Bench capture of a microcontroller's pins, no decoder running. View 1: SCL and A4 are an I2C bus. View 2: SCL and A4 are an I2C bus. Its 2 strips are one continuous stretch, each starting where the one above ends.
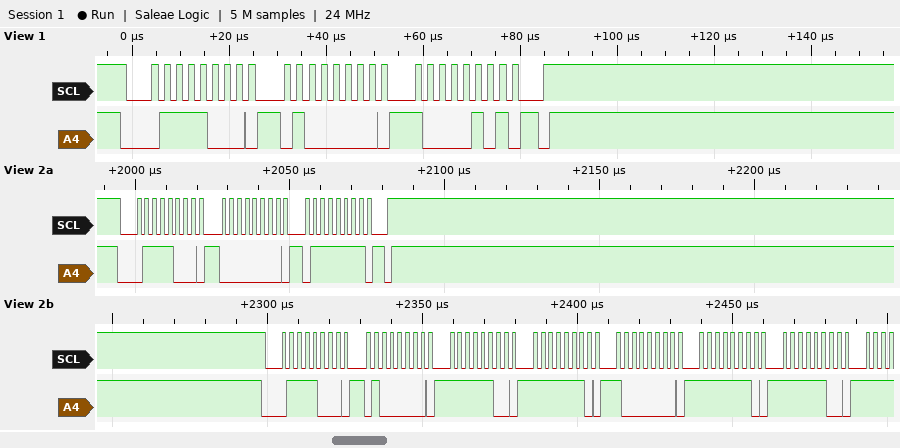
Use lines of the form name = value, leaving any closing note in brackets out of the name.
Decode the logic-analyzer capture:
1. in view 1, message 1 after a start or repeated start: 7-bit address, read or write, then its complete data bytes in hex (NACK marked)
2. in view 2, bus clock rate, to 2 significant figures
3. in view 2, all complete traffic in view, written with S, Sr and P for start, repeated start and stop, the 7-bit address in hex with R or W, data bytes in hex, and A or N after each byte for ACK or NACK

in view 1, message 1 after a start or repeated start: 7-bit address, read or write, then its complete data bytes in hex = 0x3C write: 40 85
in view 2, bus clock rate, to 2 significant figures = 400 kHz
in view 2, all complete traffic in view, written with S, Sr and P for start, repeated start and stop, the 7-bit address in hex with R or W, data bytes in hex, and A or N after each byte for ACK or NACK = S 3CW A 00 A 7F A P S 3CW A 40 A FC A FE A 80 A FE A FC A
